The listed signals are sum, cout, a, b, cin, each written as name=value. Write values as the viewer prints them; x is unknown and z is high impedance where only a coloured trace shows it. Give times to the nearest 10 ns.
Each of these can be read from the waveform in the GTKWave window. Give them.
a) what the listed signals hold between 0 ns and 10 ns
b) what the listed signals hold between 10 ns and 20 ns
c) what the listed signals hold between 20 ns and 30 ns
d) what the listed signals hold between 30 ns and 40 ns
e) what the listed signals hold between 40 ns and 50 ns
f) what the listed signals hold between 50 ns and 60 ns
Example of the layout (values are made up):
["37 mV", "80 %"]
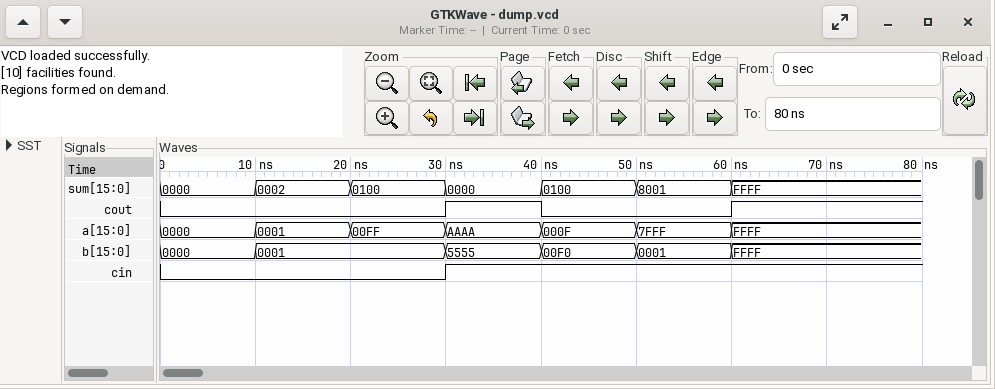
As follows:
["sum=0000, cout=0, a=0000, b=0000, cin=0", "sum=0002, cout=0, a=0001, b=0001, cin=0", "sum=0100, cout=0, a=00FF, b=0001, cin=0", "sum=0000, cout=1, a=AAAA, b=5555, cin=1", "sum=0100, cout=0, a=000F, b=00F0, cin=1", "sum=8001, cout=0, a=7FFF, b=0001, cin=1"]
